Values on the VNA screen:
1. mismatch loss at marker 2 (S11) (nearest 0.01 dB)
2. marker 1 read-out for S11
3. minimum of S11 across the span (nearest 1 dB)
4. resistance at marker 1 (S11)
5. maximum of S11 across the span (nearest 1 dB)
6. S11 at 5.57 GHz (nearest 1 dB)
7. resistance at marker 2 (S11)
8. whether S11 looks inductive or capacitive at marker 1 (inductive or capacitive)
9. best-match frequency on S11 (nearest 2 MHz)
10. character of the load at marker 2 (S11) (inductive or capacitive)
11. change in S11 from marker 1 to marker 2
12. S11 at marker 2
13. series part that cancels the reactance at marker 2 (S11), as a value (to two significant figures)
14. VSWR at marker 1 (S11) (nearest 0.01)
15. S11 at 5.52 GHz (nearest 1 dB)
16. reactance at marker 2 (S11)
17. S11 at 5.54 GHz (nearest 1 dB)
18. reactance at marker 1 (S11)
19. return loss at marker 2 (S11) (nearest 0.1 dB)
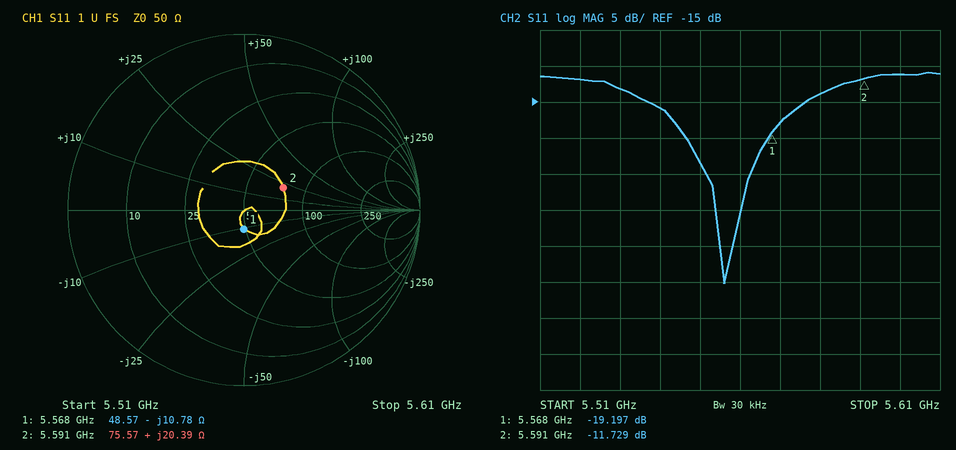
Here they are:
0.30 dB
-19.197 dB
-40 dB
48.57 Ω
-11 dB
-18 dB
75.57 Ω
capacitive
5.556 GHz
inductive
7.468 dB
-11.729 dB
1.4 pF
1.25
-12 dB
+20.39 Ω
-16 dB
-10.78 Ω
11.8 dB
